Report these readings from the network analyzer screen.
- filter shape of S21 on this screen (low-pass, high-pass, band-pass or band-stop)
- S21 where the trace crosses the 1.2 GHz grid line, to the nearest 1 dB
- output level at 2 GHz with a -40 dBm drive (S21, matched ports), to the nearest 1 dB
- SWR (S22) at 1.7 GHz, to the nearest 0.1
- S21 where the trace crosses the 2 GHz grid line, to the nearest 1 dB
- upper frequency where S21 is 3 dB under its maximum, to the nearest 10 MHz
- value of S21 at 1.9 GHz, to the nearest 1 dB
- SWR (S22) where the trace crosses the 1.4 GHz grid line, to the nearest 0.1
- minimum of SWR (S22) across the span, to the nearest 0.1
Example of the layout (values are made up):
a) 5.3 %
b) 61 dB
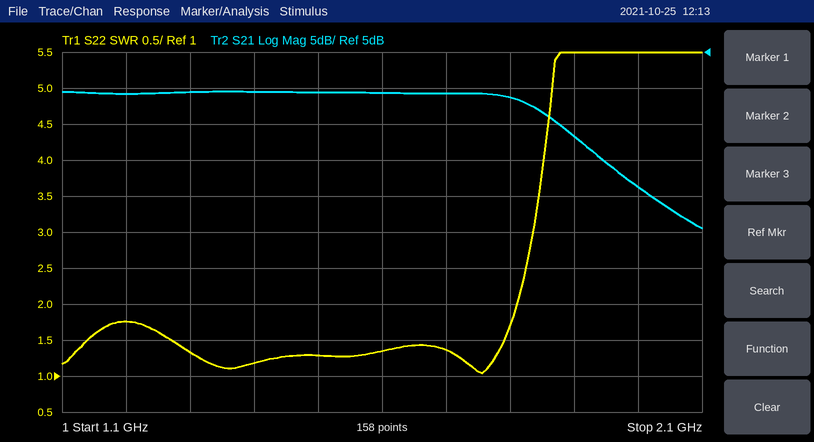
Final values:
a) low-pass
b) -1 dB
c) -54 dBm
d) 1.4
e) -14 dB
f) 1.85 GHz
g) -7 dB
h) 1.2
i) 1.0
